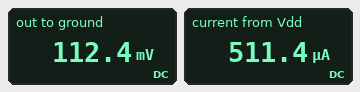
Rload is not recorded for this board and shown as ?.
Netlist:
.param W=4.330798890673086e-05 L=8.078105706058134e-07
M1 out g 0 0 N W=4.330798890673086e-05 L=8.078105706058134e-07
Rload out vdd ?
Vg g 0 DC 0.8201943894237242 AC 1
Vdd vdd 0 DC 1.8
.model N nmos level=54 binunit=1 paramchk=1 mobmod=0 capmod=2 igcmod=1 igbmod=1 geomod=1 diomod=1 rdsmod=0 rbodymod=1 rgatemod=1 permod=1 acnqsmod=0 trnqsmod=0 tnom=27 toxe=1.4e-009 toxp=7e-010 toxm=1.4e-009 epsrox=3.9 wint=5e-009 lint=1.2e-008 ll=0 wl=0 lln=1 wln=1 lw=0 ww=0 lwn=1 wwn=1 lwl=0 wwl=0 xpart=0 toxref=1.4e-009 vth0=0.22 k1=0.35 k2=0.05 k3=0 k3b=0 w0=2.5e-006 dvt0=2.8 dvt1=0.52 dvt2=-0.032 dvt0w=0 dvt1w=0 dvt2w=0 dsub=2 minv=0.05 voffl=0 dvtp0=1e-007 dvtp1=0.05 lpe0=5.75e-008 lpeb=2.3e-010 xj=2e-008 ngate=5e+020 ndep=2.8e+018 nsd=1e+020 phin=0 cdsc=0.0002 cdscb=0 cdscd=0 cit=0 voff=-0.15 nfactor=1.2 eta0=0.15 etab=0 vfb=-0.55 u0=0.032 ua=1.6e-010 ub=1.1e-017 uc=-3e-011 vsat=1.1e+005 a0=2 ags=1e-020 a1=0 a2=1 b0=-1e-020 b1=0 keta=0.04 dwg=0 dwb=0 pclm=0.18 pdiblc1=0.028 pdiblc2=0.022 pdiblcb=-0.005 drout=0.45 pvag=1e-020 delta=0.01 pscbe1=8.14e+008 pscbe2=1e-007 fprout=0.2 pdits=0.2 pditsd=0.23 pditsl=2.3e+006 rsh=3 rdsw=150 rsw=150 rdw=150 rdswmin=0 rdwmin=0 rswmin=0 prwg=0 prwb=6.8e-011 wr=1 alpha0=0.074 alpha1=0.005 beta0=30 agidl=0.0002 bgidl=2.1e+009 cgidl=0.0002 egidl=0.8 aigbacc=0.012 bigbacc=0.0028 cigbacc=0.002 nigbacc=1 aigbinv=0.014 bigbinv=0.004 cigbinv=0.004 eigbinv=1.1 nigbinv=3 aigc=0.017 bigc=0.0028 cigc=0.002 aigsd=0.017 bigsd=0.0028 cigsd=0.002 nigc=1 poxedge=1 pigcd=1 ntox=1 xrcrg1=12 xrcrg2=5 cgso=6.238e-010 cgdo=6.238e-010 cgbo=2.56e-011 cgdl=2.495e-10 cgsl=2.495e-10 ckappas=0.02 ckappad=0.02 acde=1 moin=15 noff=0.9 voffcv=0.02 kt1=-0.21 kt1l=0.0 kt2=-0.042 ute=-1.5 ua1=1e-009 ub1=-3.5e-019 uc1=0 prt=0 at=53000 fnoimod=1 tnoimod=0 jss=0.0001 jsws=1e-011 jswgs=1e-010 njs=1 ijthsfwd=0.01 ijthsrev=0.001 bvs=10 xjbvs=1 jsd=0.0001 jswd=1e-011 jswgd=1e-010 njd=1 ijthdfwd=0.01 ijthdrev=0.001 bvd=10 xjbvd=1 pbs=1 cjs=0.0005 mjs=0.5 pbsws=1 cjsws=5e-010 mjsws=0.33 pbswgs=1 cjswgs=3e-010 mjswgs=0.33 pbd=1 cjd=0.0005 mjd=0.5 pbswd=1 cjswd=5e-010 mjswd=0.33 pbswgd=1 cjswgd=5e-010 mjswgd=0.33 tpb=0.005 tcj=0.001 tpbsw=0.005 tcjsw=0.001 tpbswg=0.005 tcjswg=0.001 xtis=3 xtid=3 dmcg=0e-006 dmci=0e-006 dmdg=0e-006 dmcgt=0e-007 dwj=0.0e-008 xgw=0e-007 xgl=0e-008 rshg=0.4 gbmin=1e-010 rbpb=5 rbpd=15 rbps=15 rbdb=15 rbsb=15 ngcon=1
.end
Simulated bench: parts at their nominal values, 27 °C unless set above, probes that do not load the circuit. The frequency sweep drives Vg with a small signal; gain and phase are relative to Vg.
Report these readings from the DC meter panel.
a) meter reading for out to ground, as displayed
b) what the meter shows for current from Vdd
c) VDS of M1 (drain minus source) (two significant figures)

112.4 mV
511.4 µA
110 mV
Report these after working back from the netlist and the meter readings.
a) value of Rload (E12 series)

3.3 kΩ
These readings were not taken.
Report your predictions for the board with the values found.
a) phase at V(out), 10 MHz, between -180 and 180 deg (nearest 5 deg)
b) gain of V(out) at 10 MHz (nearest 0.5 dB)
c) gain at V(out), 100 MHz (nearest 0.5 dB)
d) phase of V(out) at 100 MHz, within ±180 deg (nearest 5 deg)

170 deg
-23.5 dB
-18.5 dB
120 deg
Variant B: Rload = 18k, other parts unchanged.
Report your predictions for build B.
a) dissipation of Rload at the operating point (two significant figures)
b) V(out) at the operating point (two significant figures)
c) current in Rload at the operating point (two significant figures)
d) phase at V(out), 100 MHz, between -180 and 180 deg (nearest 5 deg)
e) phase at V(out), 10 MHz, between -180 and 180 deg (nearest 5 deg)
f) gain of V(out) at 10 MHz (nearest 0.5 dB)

180 µW
19 mV
99 µA
90 deg
125 deg
-39.5 dB
